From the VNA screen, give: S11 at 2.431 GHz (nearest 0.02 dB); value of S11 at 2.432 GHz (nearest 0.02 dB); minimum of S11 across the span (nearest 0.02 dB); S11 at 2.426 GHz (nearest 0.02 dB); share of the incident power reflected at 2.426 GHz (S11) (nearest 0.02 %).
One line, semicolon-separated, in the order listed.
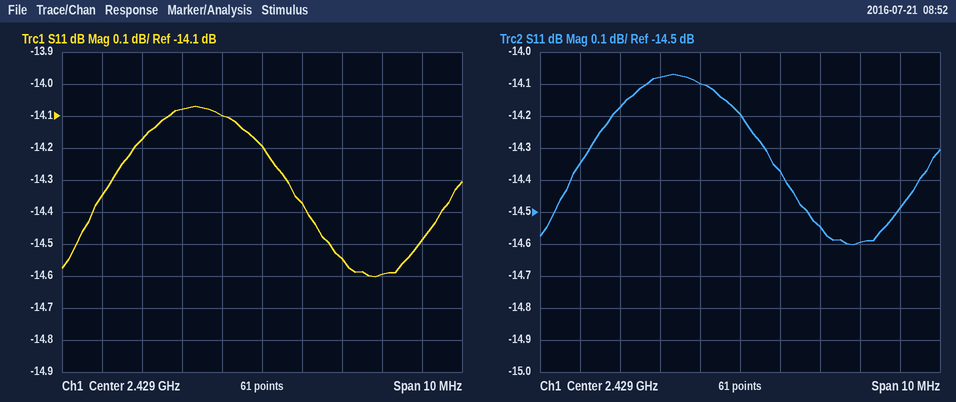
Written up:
-14.54 dB; -14.60 dB; -14.60 dB; -14.18 dB; 3.82 %
